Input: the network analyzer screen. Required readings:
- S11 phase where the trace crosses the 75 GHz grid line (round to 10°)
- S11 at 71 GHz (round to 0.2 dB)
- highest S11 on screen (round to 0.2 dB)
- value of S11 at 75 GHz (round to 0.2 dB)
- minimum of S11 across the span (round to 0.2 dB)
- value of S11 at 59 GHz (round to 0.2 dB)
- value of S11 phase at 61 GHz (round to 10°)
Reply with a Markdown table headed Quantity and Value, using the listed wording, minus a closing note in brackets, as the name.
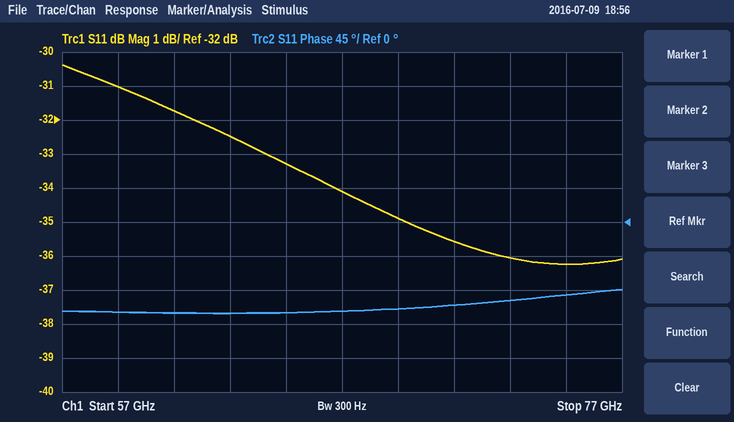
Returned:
| Quantity | Value |
|---|---|
| S11 phase where the trace crosses the 75 GHz grid line | -100° |
| S11 at 71 GHz | -35.6 dB |
| highest S11 on screen | -30.4 dB |
| value of S11 at 75 GHz | -36.2 dB |
| minimum of S11 across the span | -36.2 dB |
| value of S11 at 59 GHz | -31.0 dB |
| value of S11 phase at 61 GHz | -120° |
